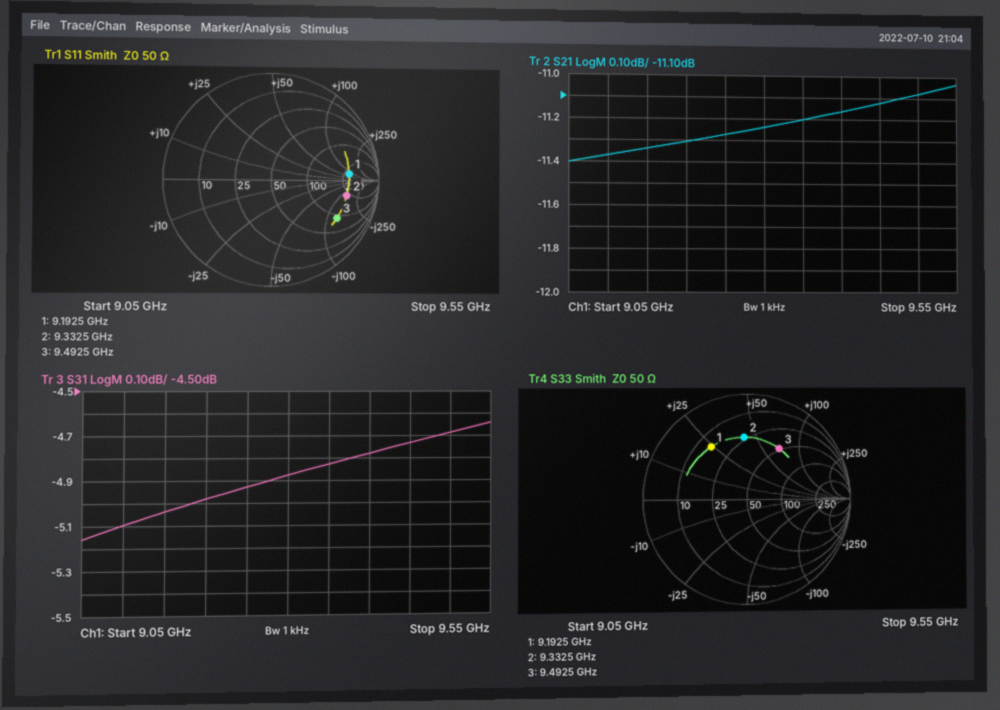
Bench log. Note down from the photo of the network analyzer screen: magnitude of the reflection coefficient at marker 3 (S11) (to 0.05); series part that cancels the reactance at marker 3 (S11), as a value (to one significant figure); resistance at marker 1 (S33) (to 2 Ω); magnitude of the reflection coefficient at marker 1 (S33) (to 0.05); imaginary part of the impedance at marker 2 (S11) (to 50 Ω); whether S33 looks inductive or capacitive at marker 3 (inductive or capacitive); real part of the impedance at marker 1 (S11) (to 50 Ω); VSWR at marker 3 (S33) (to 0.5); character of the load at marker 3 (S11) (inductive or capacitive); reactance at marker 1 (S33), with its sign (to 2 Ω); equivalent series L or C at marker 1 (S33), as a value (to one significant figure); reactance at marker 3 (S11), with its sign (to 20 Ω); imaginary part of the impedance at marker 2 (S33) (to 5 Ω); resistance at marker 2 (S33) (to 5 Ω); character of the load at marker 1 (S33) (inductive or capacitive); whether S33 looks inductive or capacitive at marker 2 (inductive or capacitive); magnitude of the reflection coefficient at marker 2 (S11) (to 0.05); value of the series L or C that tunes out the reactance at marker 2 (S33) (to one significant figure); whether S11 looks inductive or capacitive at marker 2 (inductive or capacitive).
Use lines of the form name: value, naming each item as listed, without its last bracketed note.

magnitude of the reflection coefficient at marker 3 (S11): 0.70
series part that cancels the reactance at marker 3 (S11), as a value: 2 nH
resistance at marker 1 (S33): 16 Ω
magnitude of the reflection coefficient at marker 1 (S33): 0.60
imaginary part of the impedance at marker 2 (S11): -150 Ω
whether S33 looks inductive or capacitive at marker 3: inductive
real part of the impedance at marker 1 (S11): 300 Ω
VSWR at marker 3 (S33): 3.5
character of the load at marker 3 (S11): capacitive
reactance at marker 1 (S33), with its sign: +24 Ω
equivalent series L or C at marker 1 (S33), as a value: 400 pH
reactance at marker 3 (S11), with its sign: -120 Ω
imaginary part of the impedance at marker 2 (S33): +40 Ω
resistance at marker 2 (S33): 25 Ω
character of the load at marker 1 (S33): inductive
whether S33 looks inductive or capacitive at marker 2: inductive
magnitude of the reflection coefficient at marker 2 (S11): 0.70
value of the series L or C that tunes out the reactance at marker 2 (S33): 400 fF
whether S11 looks inductive or capacitive at marker 2: capacitive
